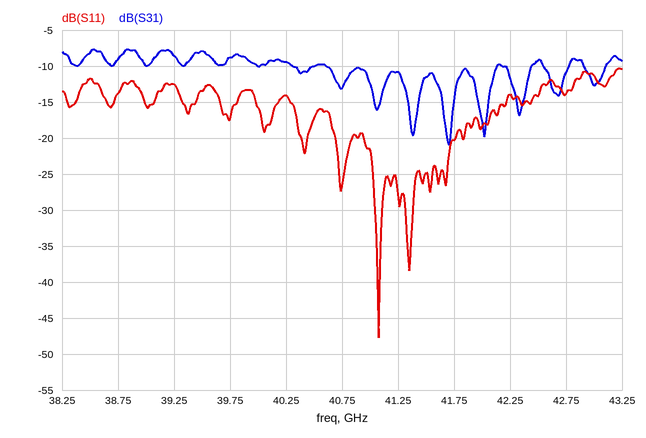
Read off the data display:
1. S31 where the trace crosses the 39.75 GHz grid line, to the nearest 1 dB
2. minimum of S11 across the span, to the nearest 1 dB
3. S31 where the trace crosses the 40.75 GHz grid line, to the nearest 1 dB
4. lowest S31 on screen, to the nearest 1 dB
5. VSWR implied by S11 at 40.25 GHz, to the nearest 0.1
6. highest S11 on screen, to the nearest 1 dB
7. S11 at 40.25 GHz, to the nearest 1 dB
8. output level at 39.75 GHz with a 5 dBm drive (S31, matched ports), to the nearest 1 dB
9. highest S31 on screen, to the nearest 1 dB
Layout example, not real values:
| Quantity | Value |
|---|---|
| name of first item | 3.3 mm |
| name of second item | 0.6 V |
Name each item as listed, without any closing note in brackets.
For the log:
| Quantity | Value |
|---|---|
| S31 where the trace crosses the 39.75 GHz grid line, to the nearest 1 dB | -9 dB |
| minimum of S11 across the span, to the nearest 1 dB | -48 dB |
| S31 where the trace crosses the 40.75 GHz grid line, to the nearest 1 dB | -13 dB |
| lowest S31 on screen, to the nearest 1 dB | -21 dB |
| VSWR implied by S11 at 40.25 GHz, to the nearest 0.1 | 1.5 |
| highest S11 on screen, to the nearest 1 dB | -10 dB |
| S11 at 40.25 GHz, to the nearest 1 dB | -14 dB |
| output level at 39.75 GHz with a 5 dBm drive (S31, matched ports), to the nearest 1 dB | -4 dBm |
| highest S31 on screen, to the nearest 1 dB | -8 dB |
